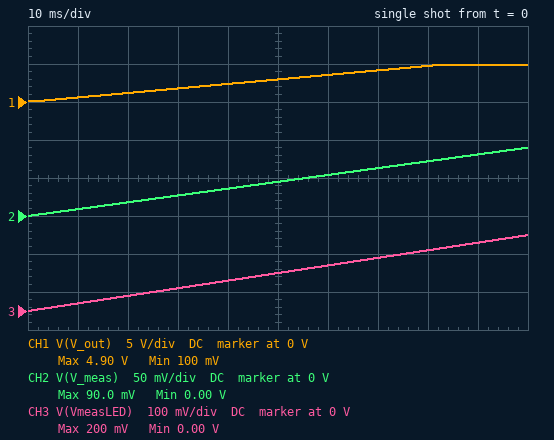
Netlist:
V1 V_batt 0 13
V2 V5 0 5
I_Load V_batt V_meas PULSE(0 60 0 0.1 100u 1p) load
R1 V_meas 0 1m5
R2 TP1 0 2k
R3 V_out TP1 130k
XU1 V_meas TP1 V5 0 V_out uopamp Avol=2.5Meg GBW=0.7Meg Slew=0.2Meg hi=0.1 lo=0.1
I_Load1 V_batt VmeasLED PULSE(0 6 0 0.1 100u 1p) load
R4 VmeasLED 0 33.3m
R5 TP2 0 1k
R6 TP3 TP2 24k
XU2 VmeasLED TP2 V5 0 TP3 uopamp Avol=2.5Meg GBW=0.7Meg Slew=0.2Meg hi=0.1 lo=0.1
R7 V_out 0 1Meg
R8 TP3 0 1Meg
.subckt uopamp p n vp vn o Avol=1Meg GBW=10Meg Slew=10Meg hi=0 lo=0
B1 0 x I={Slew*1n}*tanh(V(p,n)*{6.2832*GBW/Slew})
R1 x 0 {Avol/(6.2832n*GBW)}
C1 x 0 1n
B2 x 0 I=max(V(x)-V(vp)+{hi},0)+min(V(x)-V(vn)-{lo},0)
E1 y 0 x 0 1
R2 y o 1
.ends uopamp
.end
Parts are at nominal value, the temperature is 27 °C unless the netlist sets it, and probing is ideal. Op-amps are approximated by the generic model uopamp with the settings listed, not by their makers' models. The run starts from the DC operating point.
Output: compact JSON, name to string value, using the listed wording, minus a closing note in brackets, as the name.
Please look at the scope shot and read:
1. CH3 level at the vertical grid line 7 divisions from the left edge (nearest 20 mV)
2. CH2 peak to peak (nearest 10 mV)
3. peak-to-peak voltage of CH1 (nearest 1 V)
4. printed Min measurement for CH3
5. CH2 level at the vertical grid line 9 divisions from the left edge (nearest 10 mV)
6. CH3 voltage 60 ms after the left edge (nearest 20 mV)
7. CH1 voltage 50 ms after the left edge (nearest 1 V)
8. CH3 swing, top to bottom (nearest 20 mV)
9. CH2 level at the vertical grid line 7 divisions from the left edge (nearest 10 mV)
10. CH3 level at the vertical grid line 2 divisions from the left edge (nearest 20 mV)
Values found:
{"CH3 level at the vertical grid line 7 divisions from the left edge": "140 mV", "CH2 peak to peak": "90 mV", "peak-to-peak voltage of CH1": "5 V", "printed Min measurement for CH3": "0.00 V", "CH2 level at the vertical grid line 9 divisions from the left edge": "80 mV", "CH3 voltage 60 ms after the left edge": "120 mV", "CH1 voltage 50 ms after the left edge": "3 V", "CH3 swing, top to bottom": "200 mV", "CH2 level at the vertical grid line 7 divisions from the left edge": "60 mV", "CH3 level at the vertical grid line 2 divisions from the left edge": "40 mV"}
